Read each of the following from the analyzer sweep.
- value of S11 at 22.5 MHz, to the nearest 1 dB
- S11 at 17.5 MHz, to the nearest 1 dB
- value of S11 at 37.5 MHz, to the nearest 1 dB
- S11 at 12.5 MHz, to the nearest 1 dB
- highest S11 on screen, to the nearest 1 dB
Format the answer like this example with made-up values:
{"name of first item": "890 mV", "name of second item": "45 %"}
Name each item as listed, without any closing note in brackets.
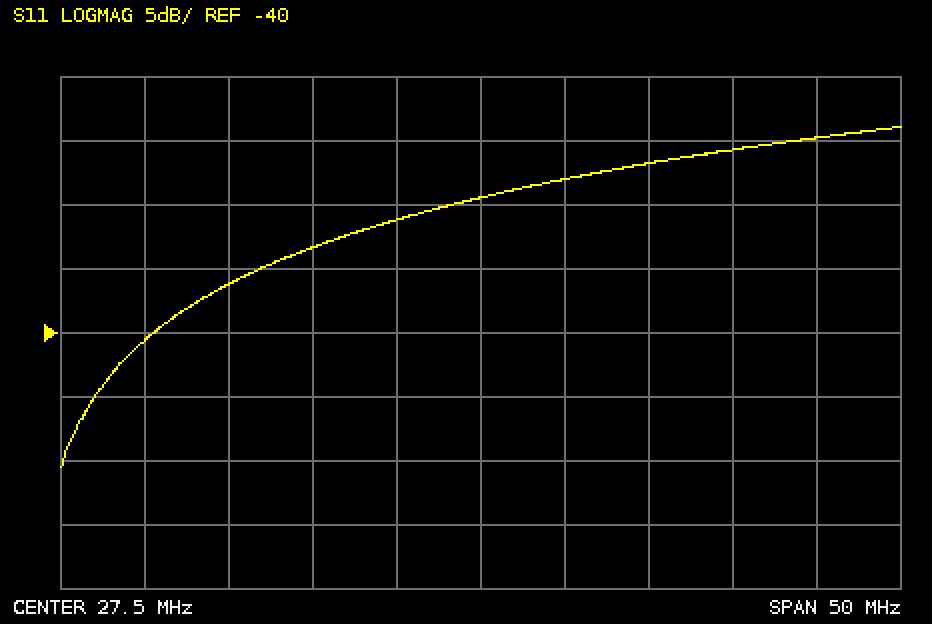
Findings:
{"value of S11 at 22.5 MHz, to the nearest 1 dB": "-31 dB", "S11 at 17.5 MHz, to the nearest 1 dB": "-33 dB", "value of S11 at 37.5 MHz, to the nearest 1 dB": "-27 dB", "S11 at 12.5 MHz, to the nearest 1 dB": "-36 dB", "highest S11 on screen, to the nearest 1 dB": "-24 dB"}
